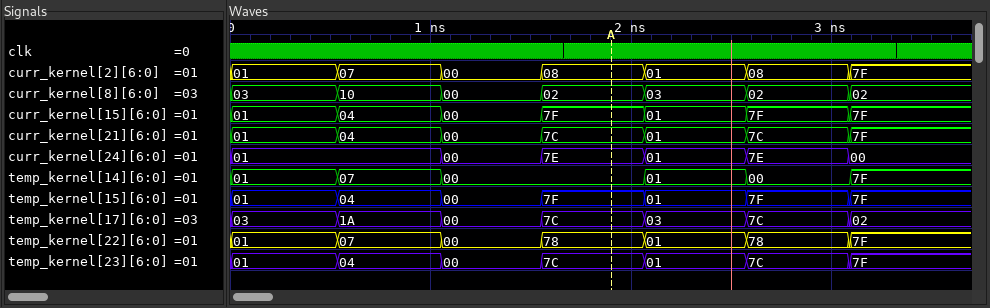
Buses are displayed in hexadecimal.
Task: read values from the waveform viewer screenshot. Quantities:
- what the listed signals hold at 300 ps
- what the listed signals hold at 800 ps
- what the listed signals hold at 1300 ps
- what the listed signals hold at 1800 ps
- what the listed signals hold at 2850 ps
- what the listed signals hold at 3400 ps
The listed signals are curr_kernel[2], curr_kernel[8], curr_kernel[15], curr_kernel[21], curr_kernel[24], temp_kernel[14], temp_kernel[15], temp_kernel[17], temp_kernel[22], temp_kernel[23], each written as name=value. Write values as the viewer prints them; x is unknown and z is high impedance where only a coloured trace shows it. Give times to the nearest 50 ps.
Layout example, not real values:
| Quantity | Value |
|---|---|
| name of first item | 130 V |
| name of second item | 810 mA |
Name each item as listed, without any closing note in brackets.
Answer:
| Quantity | Value |
|---|---|
| what the listed signals hold at 300 ps | curr_kernel[2]=01, curr_kernel[8]=03, curr_kernel[15]=01, curr_kernel[21]=01, curr_kernel[24]=01, temp_kernel[14]=01, temp_kernel[15]=01, temp_kernel[17]=03, temp_kernel[22]=01, temp_kernel[23]=01 |
| what the listed signals hold at 800 ps | curr_kernel[2]=07, curr_kernel[8]=10, curr_kernel[15]=04, curr_kernel[21]=04, curr_kernel[24]=01, temp_kernel[14]=07, temp_kernel[15]=04, temp_kernel[17]=1A, temp_kernel[22]=07, temp_kernel[23]=04 |
| what the listed signals hold at 1300 ps | curr_kernel[2]=00, curr_kernel[8]=00, curr_kernel[15]=00, curr_kernel[21]=00, curr_kernel[24]=00, temp_kernel[14]=00, temp_kernel[15]=00, temp_kernel[17]=00, temp_kernel[22]=00, temp_kernel[23]=00 |
| what the listed signals hold at 1800 ps | curr_kernel[2]=08, curr_kernel[8]=02, curr_kernel[15]=7F, curr_kernel[21]=7C, curr_kernel[24]=7E, temp_kernel[14]=00, temp_kernel[15]=7F, temp_kernel[17]=7C, temp_kernel[22]=78, temp_kernel[23]=7C |
| what the listed signals hold at 2850 ps | curr_kernel[2]=08, curr_kernel[8]=02, curr_kernel[15]=7F, curr_kernel[21]=7C, curr_kernel[24]=7E, temp_kernel[14]=00, temp_kernel[15]=7F, temp_kernel[17]=7C, temp_kernel[22]=78, temp_kernel[23]=7C |
| what the listed signals hold at 3400 ps | curr_kernel[2]=7F, curr_kernel[8]=02, curr_kernel[15]=7F, curr_kernel[21]=7F, curr_kernel[24]=00, temp_kernel[14]=7F, temp_kernel[15]=7F, temp_kernel[17]=02, temp_kernel[22]=7F, temp_kernel[23]=7F |
